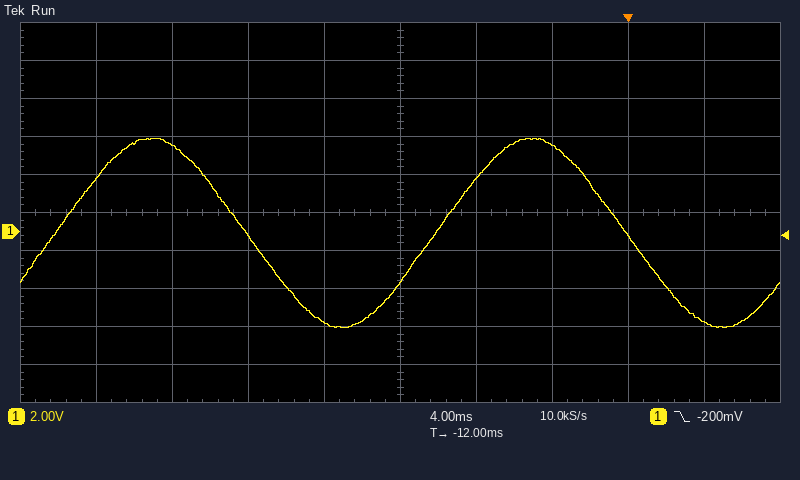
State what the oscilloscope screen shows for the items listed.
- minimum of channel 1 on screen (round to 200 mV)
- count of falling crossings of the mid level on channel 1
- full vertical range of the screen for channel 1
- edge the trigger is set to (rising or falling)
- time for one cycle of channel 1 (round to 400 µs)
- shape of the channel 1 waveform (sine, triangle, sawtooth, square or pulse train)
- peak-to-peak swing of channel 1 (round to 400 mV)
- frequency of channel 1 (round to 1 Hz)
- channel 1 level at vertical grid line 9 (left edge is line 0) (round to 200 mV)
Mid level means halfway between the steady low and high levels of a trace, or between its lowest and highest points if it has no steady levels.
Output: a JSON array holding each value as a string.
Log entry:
["-5.0 V", "2", "20 V", "falling", "20.0 ms", "sine", "10.0 V", "50 Hz", "-4.8 V"]
